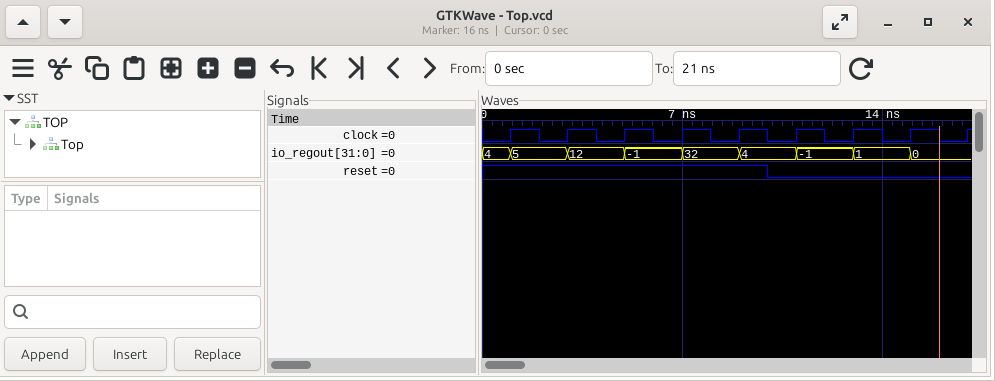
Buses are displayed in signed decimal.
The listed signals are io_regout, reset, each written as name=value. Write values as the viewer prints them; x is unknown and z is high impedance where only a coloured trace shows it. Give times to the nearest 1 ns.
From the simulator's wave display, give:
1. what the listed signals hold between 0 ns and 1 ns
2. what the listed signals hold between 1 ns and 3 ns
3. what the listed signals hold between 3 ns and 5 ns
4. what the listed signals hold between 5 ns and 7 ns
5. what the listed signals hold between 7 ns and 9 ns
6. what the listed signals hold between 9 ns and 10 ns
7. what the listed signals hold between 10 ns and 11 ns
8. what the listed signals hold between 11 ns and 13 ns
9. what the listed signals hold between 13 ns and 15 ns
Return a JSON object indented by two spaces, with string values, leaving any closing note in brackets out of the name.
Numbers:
{
  "what the listed signals hold between 0 ns and 1 ns": "io_regout=4, reset=1",
  "what the listed signals hold between 1 ns and 3 ns": "io_regout=5, reset=1",
  "what the listed signals hold between 3 ns and 5 ns": "io_regout=12, reset=1",
  "what the listed signals hold between 5 ns and 7 ns": "io_regout=-1, reset=1",
  "what the listed signals hold between 7 ns and 9 ns": "io_regout=32, reset=1",
  "what the listed signals hold between 9 ns and 10 ns": "io_regout=4, reset=1",
  "what the listed signals hold between 10 ns and 11 ns": "io_regout=4, reset=0",
  "what the listed signals hold between 11 ns and 13 ns": "io_regout=-1, reset=0",
  "what the listed signals hold between 13 ns and 15 ns": "io_regout=1, reset=0"
}
